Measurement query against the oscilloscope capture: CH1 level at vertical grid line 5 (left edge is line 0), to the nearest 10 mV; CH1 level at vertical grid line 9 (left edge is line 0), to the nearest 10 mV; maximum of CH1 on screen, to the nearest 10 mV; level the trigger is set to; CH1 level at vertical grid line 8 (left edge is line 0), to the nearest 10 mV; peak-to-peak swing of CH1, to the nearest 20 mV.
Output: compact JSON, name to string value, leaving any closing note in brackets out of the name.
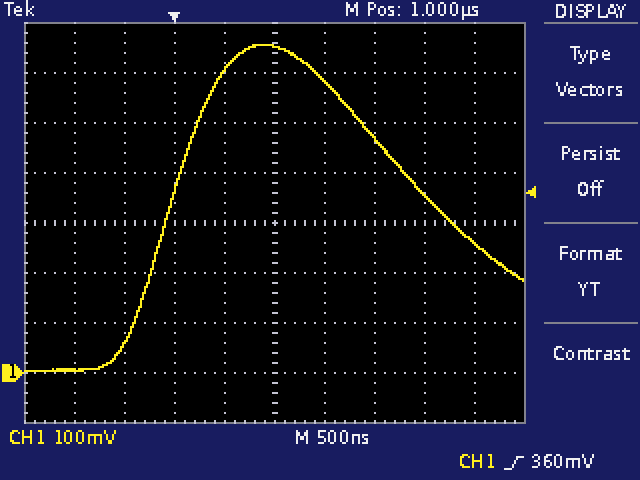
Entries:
{"CH1 level at vertical grid line 5 (left edge is line 0), to the nearest 10 mV": "650 mV", "CH1 level at vertical grid line 9 (left edge is line 0), to the nearest 10 mV": "260 mV", "maximum of CH1 on screen, to the nearest 10 mV": "660 mV", "level the trigger is set to": "360 mV", "CH1 level at vertical grid line 8 (left edge is line 0), to the nearest 10 mV": "360 mV", "peak-to-peak swing of CH1, to the nearest 20 mV": "660 mV"}
